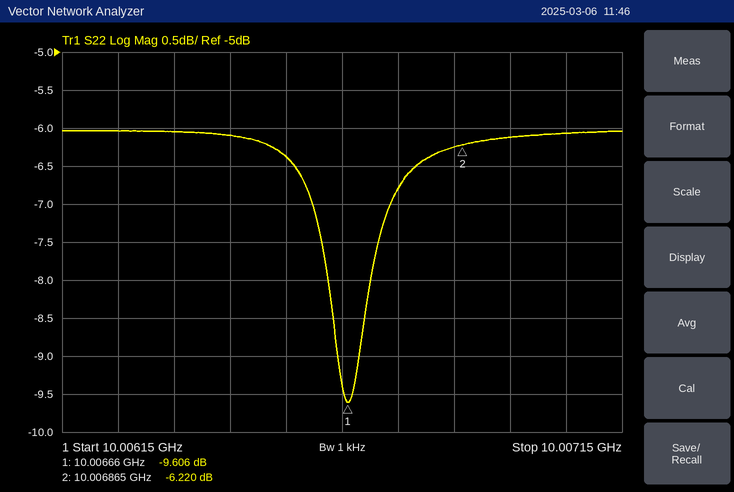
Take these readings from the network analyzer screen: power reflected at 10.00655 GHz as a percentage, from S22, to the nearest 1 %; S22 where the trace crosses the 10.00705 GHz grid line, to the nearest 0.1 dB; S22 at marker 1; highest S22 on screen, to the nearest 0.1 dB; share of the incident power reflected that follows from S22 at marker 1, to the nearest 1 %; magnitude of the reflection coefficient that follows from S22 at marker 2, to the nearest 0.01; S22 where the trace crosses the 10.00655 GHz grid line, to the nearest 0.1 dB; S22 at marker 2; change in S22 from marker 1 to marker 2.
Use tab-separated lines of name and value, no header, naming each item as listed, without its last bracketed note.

power reflected at 10.00655 GHz as a percentage, from S22, to the nearest 1 %	23 %
S22 where the trace crosses the 10.00705 GHz grid line, to the nearest 0.1 dB	-6.1 dB
S22 at marker 1	-9.606 dB
highest S22 on screen, to the nearest 0.1 dB	-6.0 dB
share of the incident power reflected that follows from S22 at marker 1, to the nearest 1 %	11 %
magnitude of the reflection coefficient that follows from S22 at marker 2, to the nearest 0.01	0.49
S22 where the trace crosses the 10.00655 GHz grid line, to the nearest 0.1 dB	-6.4 dB
S22 at marker 2	-6.220 dB
change in S22 from marker 1 to marker 2	3.386 dB
